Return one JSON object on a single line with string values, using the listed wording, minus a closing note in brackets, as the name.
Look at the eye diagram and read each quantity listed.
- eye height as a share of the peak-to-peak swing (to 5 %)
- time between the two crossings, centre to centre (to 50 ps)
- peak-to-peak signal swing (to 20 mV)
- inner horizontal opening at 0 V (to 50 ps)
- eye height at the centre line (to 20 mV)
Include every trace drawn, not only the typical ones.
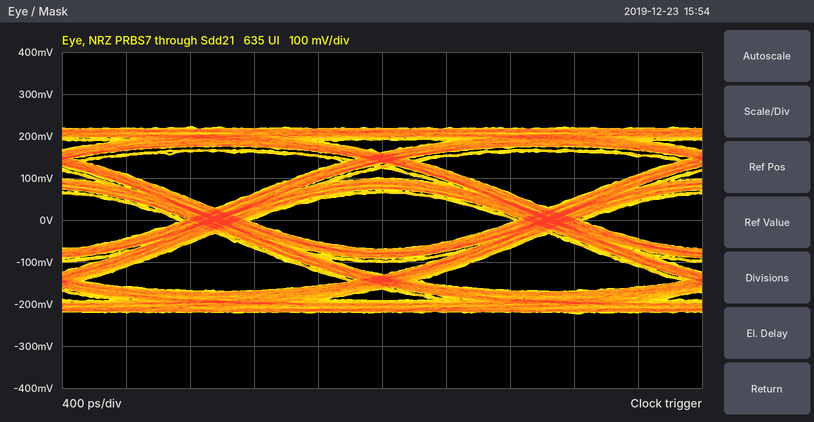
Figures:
{"eye height as a share of the peak-to-peak swing": "30 %", "time between the two crossings, centre to centre": "2.10 ns", "peak-to-peak signal swing": "440 mV", "inner horizontal opening at 0 V": "1.65 ns", "eye height at the centre line": "140 mV"}
